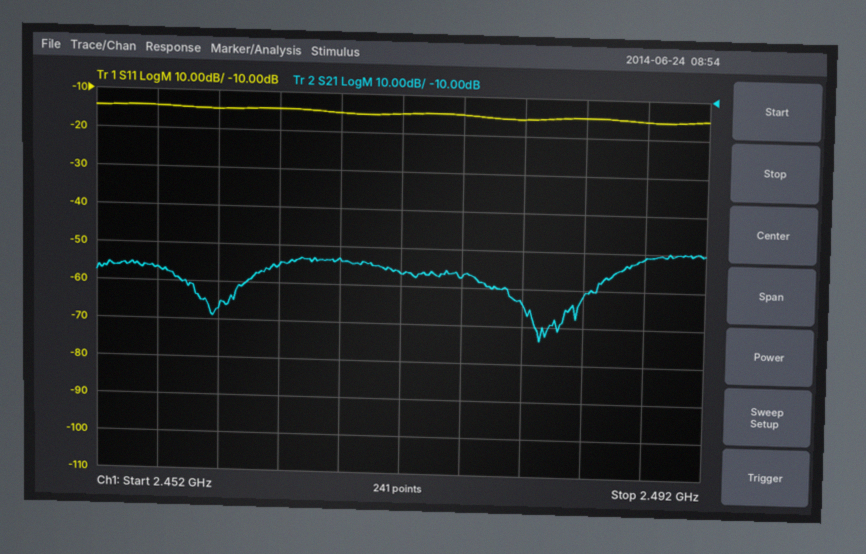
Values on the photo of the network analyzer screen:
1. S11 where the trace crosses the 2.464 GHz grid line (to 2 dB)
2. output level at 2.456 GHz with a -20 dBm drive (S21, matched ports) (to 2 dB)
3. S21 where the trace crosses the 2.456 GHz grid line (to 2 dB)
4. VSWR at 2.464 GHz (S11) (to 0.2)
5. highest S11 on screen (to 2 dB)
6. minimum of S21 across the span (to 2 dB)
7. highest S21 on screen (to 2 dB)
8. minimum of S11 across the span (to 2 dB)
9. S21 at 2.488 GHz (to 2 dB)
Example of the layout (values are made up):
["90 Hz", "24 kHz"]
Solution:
["-14 dB", "-76 dBm", "-56 dB", "1.4", "-14 dB", "-74 dB", "-50 dB", "-16 dB", "-52 dB"]
